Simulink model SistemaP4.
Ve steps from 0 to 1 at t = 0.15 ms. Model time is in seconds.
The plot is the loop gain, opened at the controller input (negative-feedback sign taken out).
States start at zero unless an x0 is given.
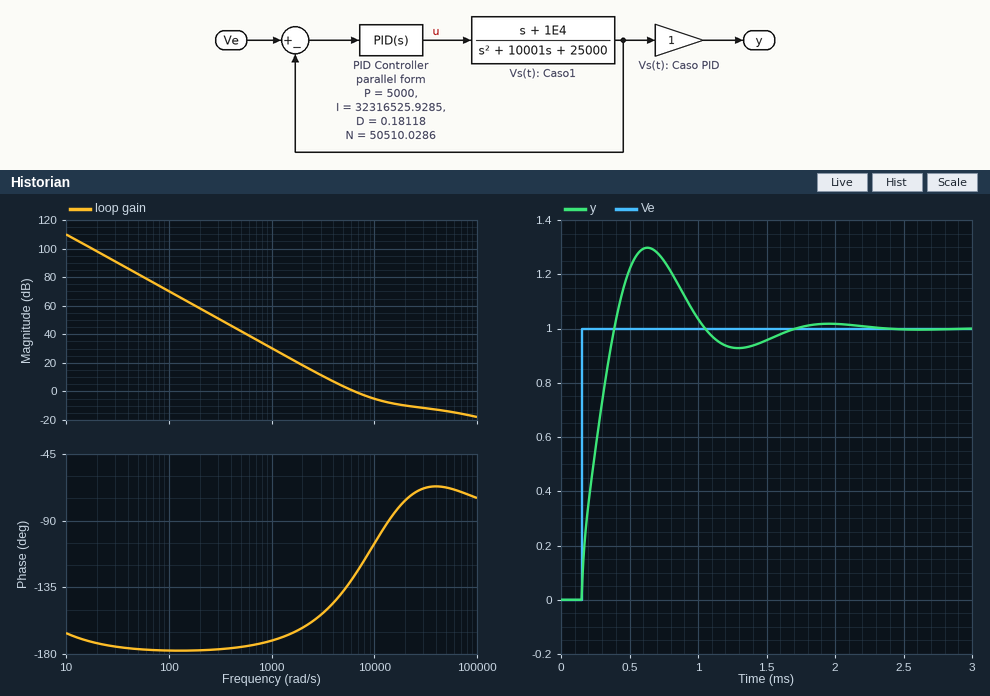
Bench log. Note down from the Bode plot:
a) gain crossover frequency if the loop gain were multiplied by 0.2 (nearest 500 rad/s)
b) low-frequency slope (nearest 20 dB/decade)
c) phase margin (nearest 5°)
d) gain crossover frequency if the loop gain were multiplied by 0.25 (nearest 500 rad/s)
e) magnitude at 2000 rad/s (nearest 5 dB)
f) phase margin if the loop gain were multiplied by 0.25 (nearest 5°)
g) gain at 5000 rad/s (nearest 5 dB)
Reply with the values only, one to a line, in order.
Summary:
2500 rad/s
-40 dB/decade
55°
3000 rad/s
20 dB
25°
5 dB
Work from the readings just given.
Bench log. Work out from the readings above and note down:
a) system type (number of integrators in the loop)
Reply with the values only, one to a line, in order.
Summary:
2
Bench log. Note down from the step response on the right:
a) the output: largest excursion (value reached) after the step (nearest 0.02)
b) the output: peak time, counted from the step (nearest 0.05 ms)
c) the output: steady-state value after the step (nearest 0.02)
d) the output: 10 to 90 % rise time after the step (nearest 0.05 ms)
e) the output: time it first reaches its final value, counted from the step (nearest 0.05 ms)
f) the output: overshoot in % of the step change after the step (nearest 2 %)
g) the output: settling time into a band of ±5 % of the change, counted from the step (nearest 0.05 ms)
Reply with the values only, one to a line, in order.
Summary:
1.30
0.50 ms
1.00
0.20 ms
0.25 ms
30 %
1.30 ms
